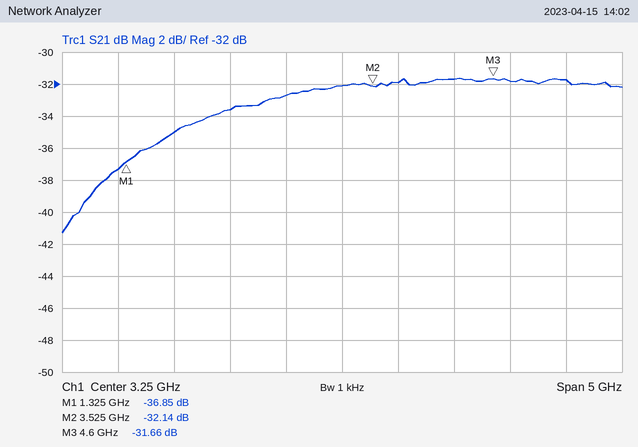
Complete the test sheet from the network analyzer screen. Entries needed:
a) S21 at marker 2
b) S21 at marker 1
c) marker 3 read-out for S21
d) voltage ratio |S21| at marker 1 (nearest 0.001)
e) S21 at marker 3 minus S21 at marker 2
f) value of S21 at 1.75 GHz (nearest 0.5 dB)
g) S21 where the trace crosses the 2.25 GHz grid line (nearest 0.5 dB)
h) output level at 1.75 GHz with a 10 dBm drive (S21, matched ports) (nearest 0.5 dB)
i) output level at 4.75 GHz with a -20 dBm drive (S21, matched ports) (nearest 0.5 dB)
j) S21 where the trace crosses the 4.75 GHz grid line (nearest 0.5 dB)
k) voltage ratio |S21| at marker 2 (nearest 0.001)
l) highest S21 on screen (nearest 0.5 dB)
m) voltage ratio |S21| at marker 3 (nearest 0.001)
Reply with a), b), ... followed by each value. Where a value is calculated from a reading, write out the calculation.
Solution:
a) -32.14 dB
b) -36.85 dB
c) -31.66 dB
d) 10^(-36.85/20) ≈ 0.014
e) -31.66 − (-32.14) = 0.48 dB
f) -35.0 dB
g) -33.5 dB
h) 10 dBm + (-35.0 dB) = -25.0 dBm
i) -20 dBm + (-32.0 dB) = -52.0 dBm
j) -32.0 dB
k) 10^(-32.14/20) ≈ 0.025
l) -31.5 dB
m) 10^(-31.66/20) ≈ 0.026
